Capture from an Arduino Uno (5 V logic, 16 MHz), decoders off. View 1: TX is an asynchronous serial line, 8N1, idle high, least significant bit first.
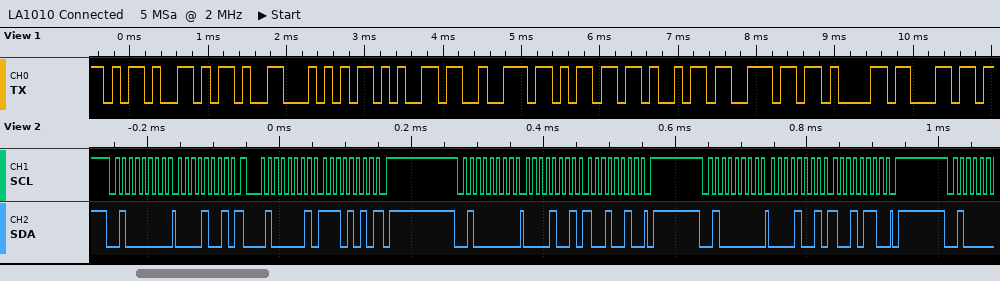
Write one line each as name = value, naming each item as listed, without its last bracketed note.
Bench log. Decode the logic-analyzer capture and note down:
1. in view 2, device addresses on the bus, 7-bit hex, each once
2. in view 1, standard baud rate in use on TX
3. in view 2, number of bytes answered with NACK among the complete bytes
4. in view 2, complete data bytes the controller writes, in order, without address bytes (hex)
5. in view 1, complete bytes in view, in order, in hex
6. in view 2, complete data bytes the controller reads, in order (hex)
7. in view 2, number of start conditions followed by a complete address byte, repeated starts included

in view 2, device addresses on the bus, 7-bit hex, each once = 0x20
in view 1, standard baud rate in use on TX = 9600 baud
in view 2, number of bytes answered with NACK among the complete bytes = 1
in view 2, complete data bytes the controller writes, in order, without address bytes = 09 09 92 09 96
in view 1, complete bytes in view, in order, in hex = 2D 2D 54 65 72 6D 69 6E 61 6C
in view 2, complete data bytes the controller reads, in order = EA
in view 2, number of start conditions followed by a complete address byte, repeated starts included = 4
